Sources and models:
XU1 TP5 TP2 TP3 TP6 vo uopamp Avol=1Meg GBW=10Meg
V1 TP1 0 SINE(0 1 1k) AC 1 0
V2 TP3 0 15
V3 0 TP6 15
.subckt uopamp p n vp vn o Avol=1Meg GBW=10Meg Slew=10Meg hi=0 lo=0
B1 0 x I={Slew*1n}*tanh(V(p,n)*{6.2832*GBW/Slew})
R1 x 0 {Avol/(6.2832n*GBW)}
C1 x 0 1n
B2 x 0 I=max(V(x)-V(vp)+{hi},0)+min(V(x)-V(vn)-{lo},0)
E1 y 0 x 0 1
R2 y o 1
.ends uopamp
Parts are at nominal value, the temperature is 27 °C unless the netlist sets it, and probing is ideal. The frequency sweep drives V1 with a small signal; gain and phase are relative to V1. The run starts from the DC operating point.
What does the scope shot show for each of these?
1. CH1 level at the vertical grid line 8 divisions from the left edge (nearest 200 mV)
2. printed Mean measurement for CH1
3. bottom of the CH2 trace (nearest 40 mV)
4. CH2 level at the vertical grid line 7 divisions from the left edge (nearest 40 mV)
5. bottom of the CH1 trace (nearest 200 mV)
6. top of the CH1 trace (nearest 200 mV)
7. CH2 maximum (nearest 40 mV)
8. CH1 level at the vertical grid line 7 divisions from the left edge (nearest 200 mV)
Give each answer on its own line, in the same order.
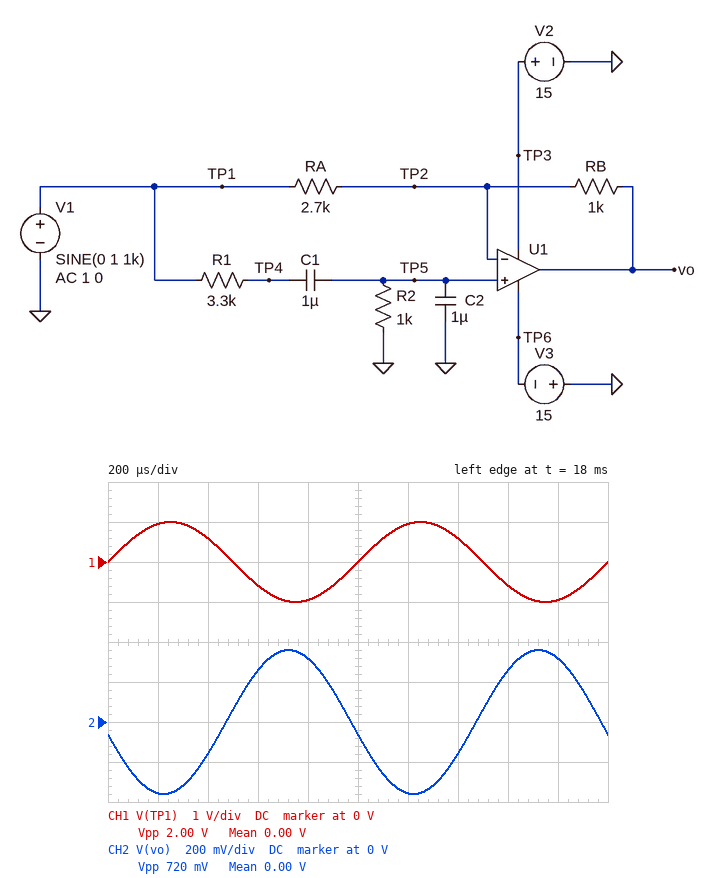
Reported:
-600 mV
0.00 V
-360 mV
-160 mV
-1.0 V
1.0 V
360 mV
600 mV
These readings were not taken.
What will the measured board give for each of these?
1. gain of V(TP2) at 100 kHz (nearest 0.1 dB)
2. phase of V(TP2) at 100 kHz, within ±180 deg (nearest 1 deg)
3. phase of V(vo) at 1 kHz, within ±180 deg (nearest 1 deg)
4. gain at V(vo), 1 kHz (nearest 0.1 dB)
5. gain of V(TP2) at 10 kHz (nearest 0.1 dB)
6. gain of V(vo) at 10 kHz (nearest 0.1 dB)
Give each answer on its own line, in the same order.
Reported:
-49.8 dB
89 deg
-170 deg
-8.9 dB
-47.0 dB
-8.6 dB
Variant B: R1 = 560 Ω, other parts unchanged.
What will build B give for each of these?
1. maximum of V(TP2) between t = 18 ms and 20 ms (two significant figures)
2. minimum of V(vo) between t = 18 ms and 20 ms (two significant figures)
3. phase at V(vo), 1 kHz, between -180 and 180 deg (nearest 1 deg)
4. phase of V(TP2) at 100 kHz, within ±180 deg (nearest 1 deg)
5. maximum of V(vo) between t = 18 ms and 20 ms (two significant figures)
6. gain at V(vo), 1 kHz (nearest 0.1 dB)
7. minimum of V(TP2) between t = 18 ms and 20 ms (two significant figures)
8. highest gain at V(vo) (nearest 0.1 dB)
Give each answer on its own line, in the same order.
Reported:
240 mV
-310 mV
-124 deg
88 deg
310 mV
-10.1 dB
-240 mV
-8.6 dB
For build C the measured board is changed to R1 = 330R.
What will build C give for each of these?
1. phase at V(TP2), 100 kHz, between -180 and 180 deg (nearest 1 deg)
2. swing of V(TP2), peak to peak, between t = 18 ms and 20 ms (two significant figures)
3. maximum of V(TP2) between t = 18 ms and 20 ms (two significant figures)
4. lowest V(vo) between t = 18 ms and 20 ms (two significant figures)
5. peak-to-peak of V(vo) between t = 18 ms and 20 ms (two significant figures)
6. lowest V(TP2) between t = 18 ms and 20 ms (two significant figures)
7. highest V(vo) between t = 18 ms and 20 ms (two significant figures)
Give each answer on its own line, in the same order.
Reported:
-88 deg
660 mV
330 mV
-290 mV
580 mV
-330 mV
290 mV
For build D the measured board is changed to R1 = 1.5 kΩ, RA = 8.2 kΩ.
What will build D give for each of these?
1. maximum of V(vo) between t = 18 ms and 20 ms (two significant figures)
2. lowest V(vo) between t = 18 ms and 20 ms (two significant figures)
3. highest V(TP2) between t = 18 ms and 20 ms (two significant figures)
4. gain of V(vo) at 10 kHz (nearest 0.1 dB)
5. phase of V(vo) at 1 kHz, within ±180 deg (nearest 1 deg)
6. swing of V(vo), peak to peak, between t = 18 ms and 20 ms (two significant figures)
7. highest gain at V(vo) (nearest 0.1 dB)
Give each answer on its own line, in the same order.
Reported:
130 mV
-130 mV
100 mV
-18.3 dB
-128 deg
270 mV
-14.0 dB
